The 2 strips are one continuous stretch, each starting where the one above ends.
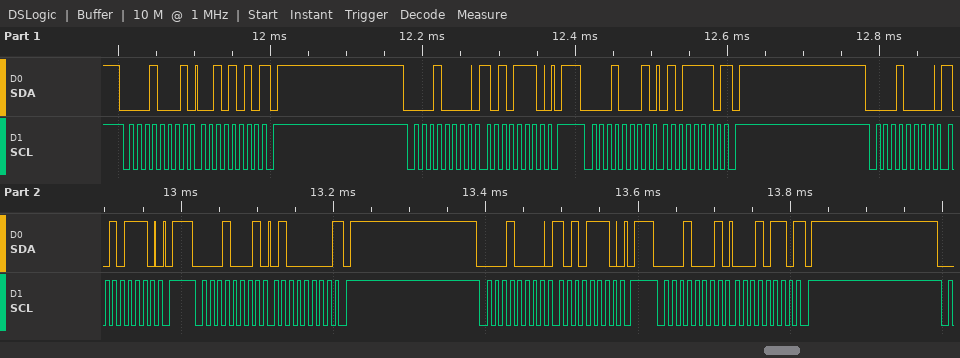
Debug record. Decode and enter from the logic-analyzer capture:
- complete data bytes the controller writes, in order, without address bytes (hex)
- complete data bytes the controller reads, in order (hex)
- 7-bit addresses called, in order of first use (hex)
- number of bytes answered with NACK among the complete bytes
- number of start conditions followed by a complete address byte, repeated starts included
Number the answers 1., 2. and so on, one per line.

1. AE AE AE
2. 2A 5E 40 16
3. 0x08
4. 4
5. 7
